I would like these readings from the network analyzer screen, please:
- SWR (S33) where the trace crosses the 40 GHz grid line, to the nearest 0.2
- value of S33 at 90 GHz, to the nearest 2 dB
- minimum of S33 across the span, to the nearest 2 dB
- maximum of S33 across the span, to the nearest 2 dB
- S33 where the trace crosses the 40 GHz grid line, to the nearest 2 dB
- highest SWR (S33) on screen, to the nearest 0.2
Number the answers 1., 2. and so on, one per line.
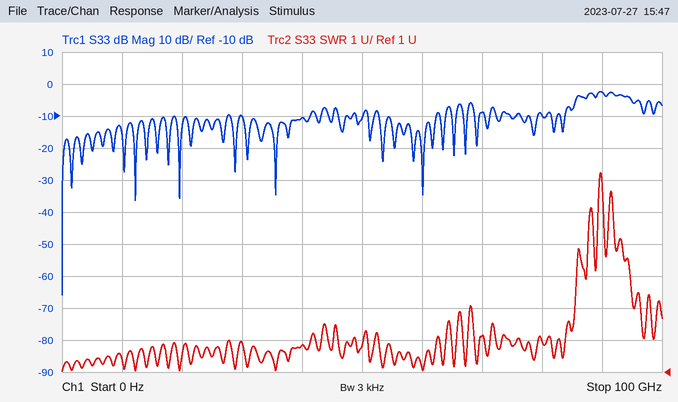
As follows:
1. 1.8
2. -2 dB
3. -66 dB
4. -2 dB
5. -10 dB
6. 7.2
